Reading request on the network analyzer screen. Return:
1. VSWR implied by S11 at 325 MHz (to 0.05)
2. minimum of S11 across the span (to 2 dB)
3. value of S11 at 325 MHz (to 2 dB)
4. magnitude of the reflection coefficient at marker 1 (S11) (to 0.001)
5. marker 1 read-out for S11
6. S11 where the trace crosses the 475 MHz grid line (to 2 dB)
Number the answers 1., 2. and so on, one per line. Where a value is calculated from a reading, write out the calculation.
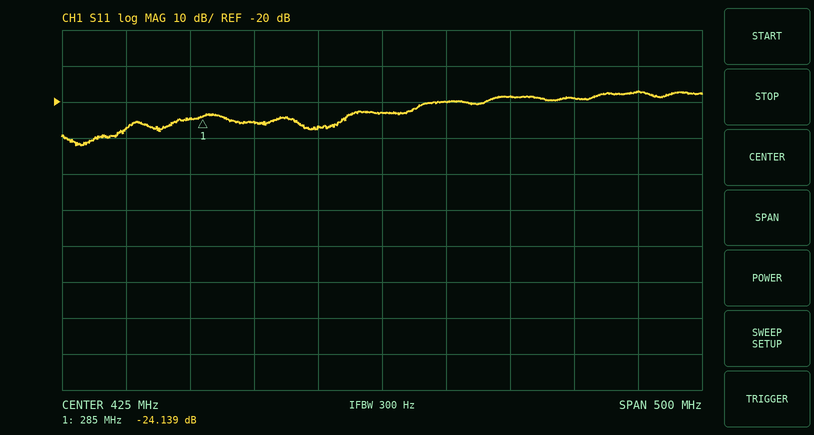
1. |Γ| = 10^(-26/20) = 0.0501; VSWR = (1 + 0.0501)/(1 − 0.0501) ≈ 1.11, so 1.10 to the nearest 0.05
2. -32 dB
3. -26 dB
4. 10^(-24.139/20) ≈ 0.062
5. -24.139 dB
6. -20 dB
